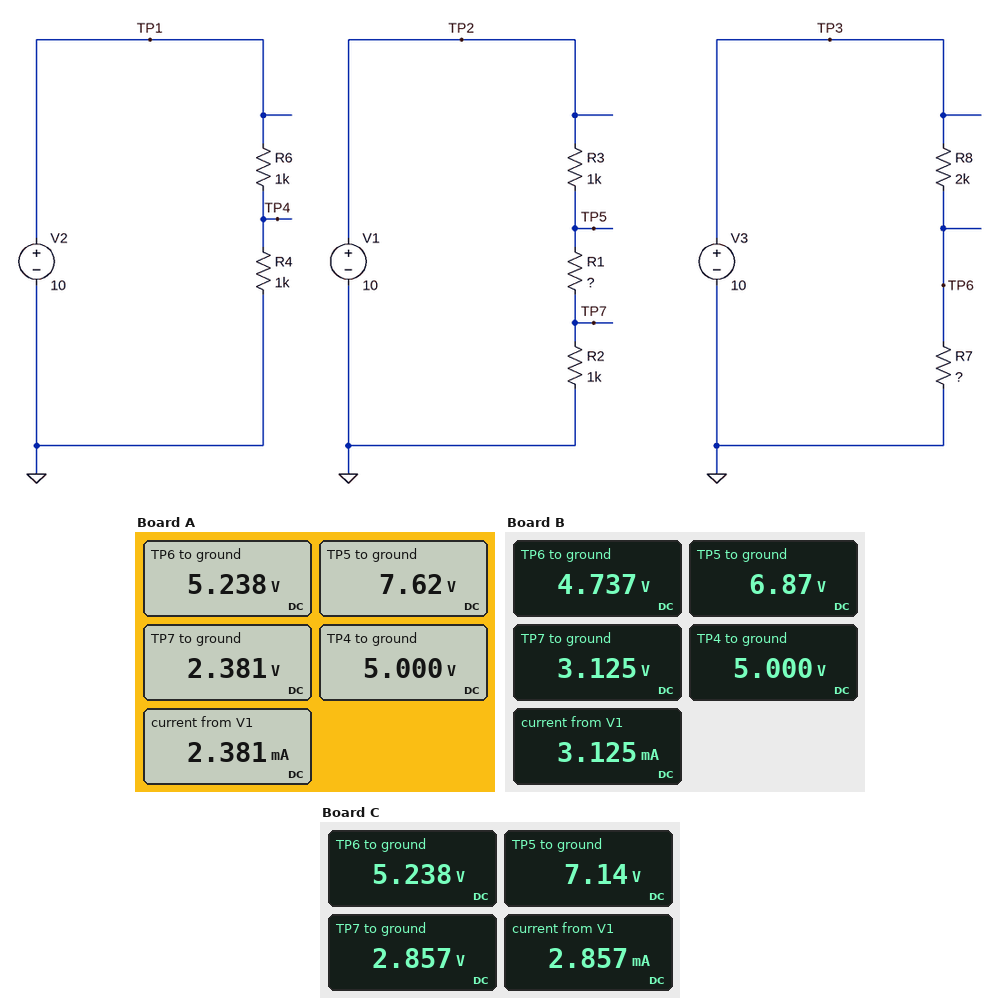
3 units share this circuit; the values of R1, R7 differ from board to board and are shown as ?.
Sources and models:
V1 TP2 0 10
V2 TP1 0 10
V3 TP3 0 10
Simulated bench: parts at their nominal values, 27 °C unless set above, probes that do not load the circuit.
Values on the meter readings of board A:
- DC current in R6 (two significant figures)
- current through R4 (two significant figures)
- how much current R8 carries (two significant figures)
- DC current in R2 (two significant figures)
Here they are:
5.0 mA
5.0 mA
2.4 mA
2.4 mA
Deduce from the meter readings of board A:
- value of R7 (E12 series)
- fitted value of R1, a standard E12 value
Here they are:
2.2 kΩ
2.2 kΩ
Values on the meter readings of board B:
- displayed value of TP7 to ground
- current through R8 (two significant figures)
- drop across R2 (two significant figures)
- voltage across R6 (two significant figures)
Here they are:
3.125 V
2.6 mA
3.1 V
5.0 V
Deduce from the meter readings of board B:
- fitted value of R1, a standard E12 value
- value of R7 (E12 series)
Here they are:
1.2 kΩ
1.8 kΩ
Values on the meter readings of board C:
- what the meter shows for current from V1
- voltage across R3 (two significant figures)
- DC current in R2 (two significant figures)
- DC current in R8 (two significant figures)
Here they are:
2.857 mA
2.9 V
2.9 mA
2.4 mA
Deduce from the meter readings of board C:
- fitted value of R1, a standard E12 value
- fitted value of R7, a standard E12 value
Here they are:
1.5 kΩ
2.2 kΩ
